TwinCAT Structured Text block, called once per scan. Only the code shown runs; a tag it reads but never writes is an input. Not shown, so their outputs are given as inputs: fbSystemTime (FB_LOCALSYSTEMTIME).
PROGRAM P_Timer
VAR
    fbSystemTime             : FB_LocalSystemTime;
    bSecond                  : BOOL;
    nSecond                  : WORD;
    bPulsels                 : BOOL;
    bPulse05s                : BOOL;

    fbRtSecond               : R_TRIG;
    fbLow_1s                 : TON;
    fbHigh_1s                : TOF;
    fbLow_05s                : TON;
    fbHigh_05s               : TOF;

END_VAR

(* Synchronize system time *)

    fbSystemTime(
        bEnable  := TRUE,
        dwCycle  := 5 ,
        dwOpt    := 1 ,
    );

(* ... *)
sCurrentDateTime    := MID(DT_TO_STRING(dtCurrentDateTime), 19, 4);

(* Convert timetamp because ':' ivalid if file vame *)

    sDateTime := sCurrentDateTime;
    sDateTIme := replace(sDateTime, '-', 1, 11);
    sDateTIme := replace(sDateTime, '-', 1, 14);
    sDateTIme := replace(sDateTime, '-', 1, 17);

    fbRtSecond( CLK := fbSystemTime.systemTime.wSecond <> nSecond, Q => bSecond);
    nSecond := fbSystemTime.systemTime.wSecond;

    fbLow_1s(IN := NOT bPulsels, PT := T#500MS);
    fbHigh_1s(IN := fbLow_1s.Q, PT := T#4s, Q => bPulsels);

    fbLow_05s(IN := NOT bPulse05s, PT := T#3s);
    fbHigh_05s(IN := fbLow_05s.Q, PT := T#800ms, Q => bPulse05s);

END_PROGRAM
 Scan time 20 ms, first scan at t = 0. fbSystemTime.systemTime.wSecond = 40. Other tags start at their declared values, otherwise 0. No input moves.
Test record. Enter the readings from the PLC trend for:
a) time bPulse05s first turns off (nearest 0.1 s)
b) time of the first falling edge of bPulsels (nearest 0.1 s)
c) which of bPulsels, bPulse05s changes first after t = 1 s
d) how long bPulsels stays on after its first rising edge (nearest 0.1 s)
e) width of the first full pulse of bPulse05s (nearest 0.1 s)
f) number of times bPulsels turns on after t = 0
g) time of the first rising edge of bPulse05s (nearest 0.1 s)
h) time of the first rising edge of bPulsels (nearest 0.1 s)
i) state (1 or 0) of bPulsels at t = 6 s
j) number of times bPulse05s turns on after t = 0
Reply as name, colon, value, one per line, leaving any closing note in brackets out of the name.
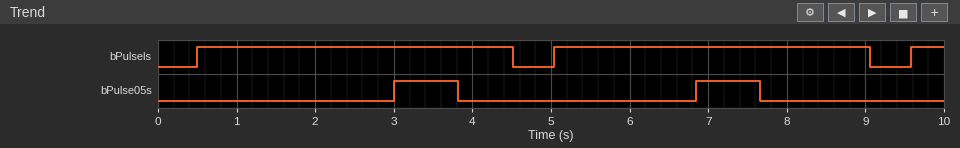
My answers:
time bPulse05s first turns off: 3.8 s
time of the first falling edge of bPulsels: 4.5 s
which of bPulsels, bPulse05s changes first after t = 1 s: bPulse05s
how long bPulsels stays on after its first rising edge: 4.0 s
width of the first full pulse of bPulse05s: 0.8 s
number of times bPulsels turns on after t = 0: 3
time of the first rising edge of bPulse05s: 3.0 s
time of the first rising edge of bPulsels: 0.5 s
state (1 or 0) of bPulsels at t = 6 s: 1
number of times bPulse05s turns on after t = 0: 2
